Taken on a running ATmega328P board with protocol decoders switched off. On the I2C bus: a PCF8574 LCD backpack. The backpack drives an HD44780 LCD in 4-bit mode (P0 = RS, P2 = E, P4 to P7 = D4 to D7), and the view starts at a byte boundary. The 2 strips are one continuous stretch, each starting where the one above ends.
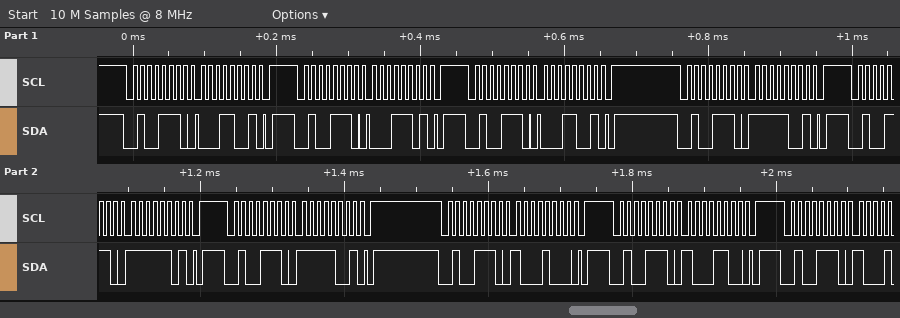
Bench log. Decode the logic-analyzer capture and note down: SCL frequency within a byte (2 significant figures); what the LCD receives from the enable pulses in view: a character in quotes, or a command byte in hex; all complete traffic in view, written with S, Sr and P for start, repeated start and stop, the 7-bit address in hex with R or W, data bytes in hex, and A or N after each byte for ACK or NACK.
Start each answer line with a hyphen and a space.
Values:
- 100 kHz
- data 0x1F
- S 27W A 19 A P S 27W A 1D A P S 27W A 19 A P S 27W A F9 A P S 27W A FD A P S 27W A F9 A P S 27W A 88 A P S 27W A 8C A P S 27W A
